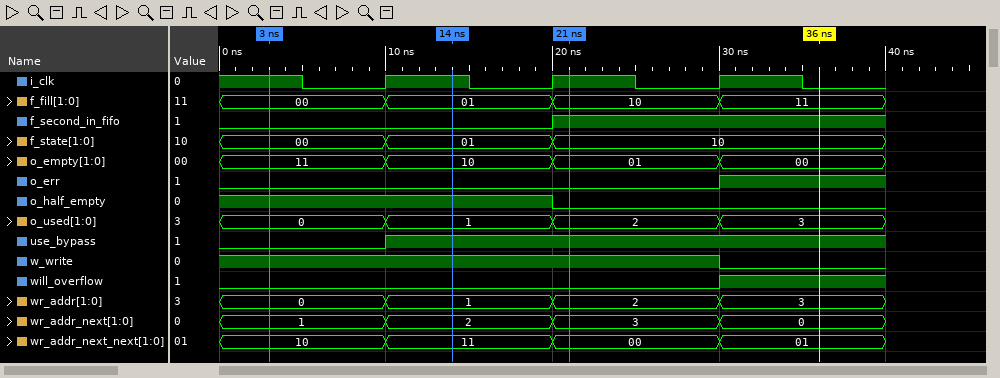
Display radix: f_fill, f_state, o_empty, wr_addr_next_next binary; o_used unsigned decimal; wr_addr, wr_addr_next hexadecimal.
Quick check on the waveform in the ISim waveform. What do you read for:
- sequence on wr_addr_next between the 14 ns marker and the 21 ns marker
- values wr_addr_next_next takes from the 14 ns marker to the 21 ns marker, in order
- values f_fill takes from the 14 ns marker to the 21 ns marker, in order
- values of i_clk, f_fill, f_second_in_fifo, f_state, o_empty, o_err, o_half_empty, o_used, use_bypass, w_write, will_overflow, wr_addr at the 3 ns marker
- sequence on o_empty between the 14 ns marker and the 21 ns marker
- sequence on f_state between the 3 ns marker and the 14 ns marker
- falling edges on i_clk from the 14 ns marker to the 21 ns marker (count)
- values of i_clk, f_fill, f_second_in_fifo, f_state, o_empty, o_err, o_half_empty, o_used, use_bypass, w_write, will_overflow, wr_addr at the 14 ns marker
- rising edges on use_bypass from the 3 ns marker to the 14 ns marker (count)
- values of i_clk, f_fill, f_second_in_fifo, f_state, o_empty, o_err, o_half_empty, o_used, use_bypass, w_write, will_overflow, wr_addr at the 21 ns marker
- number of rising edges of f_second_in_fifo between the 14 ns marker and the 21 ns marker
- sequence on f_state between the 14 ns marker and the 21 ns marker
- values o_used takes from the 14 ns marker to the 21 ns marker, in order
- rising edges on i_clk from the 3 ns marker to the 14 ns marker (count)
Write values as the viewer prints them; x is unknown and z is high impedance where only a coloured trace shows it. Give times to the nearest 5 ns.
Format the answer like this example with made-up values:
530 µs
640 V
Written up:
2, 3
11, 00
01, 10
i_clk=1, f_fill=00, f_second_in_fifo=0, f_state=00, o_empty=11, o_err=0, o_half_empty=1, o_used=0, use_bypass=0, w_write=1, will_overflow=0, wr_addr=0
10, 01
00, 01
1
i_clk=1, f_fill=01, f_second_in_fifo=0, f_state=01, o_empty=10, o_err=0, o_half_empty=1, o_used=1, use_bypass=1, w_write=1, will_overflow=0, wr_addr=1
1
i_clk=1, f_fill=10, f_second_in_fifo=1, f_state=10, o_empty=01, o_err=0, o_half_empty=0, o_used=2, use_bypass=1, w_write=1, will_overflow=0, wr_addr=2
1
01, 10
1, 2
1
